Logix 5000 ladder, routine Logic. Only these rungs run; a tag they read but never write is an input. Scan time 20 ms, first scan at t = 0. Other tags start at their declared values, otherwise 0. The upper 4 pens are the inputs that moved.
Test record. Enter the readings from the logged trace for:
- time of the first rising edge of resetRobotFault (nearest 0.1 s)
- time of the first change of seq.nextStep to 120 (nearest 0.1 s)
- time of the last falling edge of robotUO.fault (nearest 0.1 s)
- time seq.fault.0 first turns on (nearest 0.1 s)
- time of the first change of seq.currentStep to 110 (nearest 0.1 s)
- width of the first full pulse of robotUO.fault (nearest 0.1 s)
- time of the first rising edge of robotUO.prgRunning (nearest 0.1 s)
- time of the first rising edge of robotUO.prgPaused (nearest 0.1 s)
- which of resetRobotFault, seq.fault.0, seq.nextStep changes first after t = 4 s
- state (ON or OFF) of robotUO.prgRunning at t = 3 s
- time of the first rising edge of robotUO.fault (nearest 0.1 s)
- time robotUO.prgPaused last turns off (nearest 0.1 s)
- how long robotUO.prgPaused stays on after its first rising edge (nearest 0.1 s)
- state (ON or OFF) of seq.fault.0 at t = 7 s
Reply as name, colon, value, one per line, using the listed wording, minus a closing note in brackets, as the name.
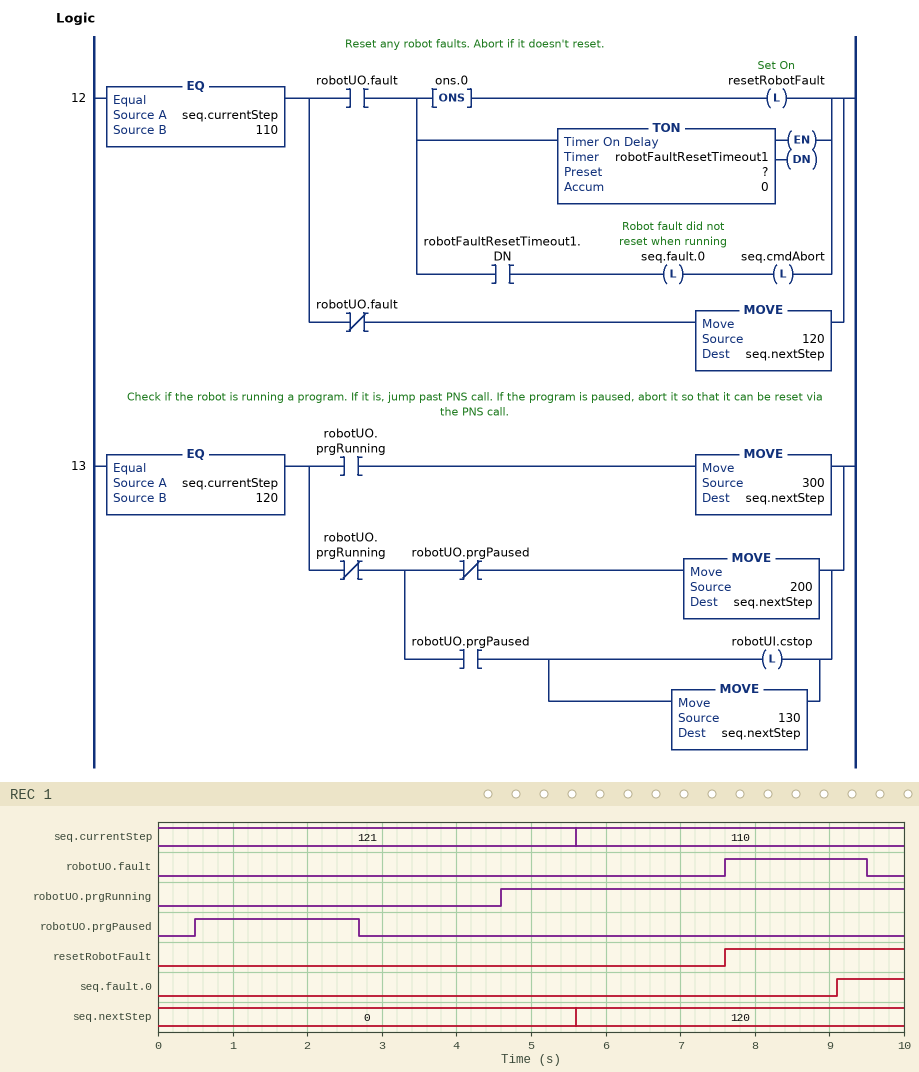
time of the first rising edge of resetRobotFault: 7.6 s
time of the first change of seq.nextStep to 120: 5.6 s
time of the last falling edge of robotUO.fault: 9.5 s
time seq.fault.0 first turns on: 9.1 s
time of the first change of seq.currentStep to 110: 5.6 s
width of the first full pulse of robotUO.fault: 1.9 s
time of the first rising edge of robotUO.prgRunning: 4.6 s
time of the first rising edge of robotUO.prgPaused: 0.5 s
which of resetRobotFault, seq.fault.0, seq.nextStep changes first after t = 4 s: seq.nextStep
state (ON or OFF) of robotUO.prgRunning at t = 3 s: OFF
time of the first rising edge of robotUO.fault: 7.6 s
time robotUO.prgPaused last turns off: 2.7 s
how long robotUO.prgPaused stays on after its first rising edge: 2.2 s
state (ON or OFF) of seq.fault.0 at t = 7 s: OFF
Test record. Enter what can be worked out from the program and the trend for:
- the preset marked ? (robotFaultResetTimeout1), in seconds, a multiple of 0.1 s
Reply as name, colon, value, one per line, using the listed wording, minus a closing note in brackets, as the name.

the preset marked ? (robotFaultResetTimeout1), in seconds, a multiple of 0.1 s: 1.5 s
